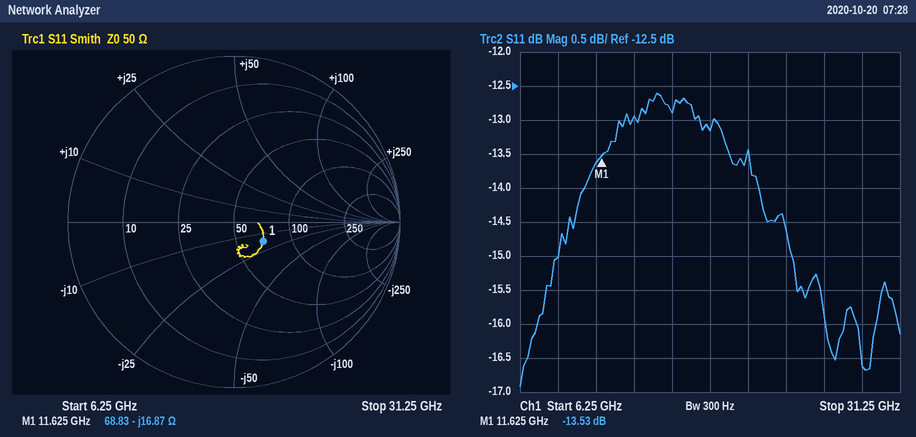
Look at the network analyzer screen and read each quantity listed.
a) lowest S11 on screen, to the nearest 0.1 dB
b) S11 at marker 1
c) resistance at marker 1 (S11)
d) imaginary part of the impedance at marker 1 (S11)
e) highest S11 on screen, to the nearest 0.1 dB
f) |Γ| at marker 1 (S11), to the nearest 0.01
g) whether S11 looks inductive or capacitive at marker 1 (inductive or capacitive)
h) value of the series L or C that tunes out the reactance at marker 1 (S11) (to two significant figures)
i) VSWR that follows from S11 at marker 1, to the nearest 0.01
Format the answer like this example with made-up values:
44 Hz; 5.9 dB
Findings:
-16.9 dB; -13.53 dB; 68.83 Ω; -16.87 Ω; -12.6 dB; 0.21; capacitive; 230 pH; 1.53
